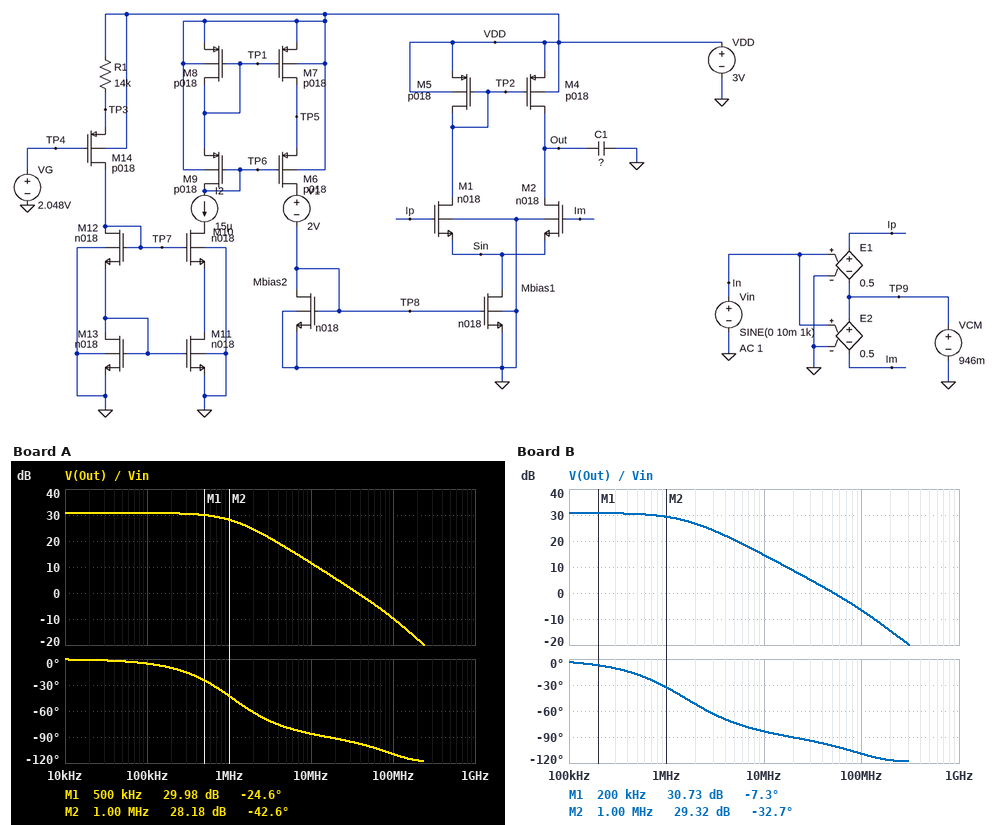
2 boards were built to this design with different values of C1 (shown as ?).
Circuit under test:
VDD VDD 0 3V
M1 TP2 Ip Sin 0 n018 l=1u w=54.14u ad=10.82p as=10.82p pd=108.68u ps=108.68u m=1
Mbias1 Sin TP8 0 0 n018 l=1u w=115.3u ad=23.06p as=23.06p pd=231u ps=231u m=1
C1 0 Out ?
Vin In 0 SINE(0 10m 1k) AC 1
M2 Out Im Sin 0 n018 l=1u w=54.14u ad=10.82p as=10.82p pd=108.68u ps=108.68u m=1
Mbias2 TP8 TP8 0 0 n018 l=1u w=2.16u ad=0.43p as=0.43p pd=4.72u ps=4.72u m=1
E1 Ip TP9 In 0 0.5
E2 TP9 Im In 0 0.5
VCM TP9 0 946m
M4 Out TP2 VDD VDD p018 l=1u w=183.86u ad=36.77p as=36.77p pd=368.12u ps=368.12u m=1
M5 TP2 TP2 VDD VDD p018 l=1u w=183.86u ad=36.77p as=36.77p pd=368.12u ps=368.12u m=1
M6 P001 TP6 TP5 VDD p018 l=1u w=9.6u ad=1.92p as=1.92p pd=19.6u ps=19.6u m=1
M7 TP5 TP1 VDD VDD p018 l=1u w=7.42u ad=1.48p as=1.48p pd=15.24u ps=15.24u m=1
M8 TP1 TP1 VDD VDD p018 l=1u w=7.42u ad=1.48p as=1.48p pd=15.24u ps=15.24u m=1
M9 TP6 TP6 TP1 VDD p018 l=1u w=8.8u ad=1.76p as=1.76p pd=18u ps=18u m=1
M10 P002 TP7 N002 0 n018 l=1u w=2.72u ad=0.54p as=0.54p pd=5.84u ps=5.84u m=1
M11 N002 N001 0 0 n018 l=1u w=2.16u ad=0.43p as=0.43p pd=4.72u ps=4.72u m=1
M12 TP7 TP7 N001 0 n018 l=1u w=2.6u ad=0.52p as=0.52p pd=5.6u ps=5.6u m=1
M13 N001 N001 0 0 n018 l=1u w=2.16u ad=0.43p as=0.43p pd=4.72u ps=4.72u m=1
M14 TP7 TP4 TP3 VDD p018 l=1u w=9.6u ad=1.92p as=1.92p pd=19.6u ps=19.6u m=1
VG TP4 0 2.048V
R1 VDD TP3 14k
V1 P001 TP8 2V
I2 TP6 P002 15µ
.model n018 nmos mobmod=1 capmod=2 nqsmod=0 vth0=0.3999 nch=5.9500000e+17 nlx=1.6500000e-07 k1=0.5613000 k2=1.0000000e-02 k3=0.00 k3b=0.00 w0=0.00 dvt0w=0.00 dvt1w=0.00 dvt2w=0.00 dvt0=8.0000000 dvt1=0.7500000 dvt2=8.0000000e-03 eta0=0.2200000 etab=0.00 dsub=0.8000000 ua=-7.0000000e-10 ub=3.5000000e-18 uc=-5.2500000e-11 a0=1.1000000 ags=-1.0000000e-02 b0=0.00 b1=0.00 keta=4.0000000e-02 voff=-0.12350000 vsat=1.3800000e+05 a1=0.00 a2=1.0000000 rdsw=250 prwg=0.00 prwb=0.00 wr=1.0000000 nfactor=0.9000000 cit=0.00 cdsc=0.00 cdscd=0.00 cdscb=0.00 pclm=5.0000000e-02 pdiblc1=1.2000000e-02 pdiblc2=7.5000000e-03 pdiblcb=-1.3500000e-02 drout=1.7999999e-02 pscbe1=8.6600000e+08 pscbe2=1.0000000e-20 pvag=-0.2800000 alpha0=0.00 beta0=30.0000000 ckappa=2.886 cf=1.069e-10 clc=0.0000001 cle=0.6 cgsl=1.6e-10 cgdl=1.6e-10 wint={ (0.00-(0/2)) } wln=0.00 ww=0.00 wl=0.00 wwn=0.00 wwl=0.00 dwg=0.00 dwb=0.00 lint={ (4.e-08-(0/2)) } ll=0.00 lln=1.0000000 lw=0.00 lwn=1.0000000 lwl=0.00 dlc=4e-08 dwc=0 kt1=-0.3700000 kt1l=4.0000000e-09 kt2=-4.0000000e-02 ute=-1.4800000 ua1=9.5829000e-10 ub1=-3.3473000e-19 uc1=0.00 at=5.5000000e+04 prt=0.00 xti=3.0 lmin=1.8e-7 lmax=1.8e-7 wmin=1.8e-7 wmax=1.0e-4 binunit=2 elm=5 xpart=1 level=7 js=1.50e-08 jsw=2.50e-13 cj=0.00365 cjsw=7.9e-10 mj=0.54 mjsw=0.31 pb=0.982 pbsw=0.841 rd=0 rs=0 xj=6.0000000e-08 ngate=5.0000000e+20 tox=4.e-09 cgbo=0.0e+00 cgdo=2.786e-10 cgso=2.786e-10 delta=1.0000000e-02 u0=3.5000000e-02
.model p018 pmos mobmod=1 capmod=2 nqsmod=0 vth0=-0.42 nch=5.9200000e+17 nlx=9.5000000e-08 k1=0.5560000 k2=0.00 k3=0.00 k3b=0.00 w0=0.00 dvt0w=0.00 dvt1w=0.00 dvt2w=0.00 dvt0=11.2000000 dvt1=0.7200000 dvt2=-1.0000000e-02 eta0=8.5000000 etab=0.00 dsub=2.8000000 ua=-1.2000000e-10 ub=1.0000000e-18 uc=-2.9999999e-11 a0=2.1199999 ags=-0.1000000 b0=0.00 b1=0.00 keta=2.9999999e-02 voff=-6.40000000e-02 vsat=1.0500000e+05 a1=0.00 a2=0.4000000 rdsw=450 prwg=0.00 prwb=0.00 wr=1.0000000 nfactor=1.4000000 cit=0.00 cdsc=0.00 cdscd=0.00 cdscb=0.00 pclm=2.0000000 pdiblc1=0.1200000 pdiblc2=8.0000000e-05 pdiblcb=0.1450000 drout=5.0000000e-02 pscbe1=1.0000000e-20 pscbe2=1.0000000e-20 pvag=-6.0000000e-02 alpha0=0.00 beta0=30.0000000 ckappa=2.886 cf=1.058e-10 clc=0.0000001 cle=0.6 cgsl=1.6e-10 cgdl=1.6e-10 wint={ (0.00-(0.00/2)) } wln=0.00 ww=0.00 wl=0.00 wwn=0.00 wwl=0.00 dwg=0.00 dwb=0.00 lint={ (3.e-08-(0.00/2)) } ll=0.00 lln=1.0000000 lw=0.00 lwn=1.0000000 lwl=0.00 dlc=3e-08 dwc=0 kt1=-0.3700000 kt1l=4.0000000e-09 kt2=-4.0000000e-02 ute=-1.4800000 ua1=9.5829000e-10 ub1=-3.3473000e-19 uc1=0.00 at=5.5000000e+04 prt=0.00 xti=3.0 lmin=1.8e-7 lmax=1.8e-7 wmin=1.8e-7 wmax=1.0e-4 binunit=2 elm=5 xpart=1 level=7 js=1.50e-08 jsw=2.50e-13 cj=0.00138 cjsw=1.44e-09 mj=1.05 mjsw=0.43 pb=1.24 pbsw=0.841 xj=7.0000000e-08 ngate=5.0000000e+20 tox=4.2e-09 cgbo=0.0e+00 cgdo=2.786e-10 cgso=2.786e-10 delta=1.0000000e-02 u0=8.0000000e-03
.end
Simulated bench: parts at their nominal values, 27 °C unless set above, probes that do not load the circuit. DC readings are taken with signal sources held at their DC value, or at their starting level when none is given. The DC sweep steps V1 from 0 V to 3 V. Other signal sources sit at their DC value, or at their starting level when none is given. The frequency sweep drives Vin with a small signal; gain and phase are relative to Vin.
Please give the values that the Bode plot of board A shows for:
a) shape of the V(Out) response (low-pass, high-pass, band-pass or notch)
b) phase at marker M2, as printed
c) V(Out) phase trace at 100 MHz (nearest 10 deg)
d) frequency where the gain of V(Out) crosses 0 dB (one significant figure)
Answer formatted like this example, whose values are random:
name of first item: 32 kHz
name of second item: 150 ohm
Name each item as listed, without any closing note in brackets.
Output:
shape of the V(Out) response: low-pass
phase at marker M2, as printed: -42.6 deg
V(Out) phase trace at 100 MHz: -110 deg
frequency where the gain of V(Out) crosses 0 dB: 40 MHz
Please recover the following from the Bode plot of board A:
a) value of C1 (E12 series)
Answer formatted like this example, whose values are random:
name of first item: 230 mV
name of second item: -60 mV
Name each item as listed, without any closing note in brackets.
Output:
value of C1: 10 pF
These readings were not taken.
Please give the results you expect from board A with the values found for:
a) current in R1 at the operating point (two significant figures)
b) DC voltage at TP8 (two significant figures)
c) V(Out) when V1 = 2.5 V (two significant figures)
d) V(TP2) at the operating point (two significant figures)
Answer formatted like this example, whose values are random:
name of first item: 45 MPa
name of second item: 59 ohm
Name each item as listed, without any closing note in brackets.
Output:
current in R1 at the operating point: 16 µA
DC voltage at TP8: 680 mV
V(Out) when V1 = 2.5 V: 2.5 V
V(TP2) at the operating point: 2.2 V
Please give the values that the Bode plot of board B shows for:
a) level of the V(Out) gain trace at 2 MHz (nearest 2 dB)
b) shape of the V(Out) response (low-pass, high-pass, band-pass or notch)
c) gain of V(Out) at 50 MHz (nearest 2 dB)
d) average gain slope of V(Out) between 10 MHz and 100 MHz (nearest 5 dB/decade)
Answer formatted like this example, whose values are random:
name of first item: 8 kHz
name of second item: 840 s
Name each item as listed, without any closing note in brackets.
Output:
level of the V(Out) gain trace at 2 MHz: 26 dB
shape of the V(Out) response: low-pass
gain of V(Out) at 50 MHz: 0 dB
average gain slope of V(Out) between 10 MHz and 100 MHz: -20 dB/decade
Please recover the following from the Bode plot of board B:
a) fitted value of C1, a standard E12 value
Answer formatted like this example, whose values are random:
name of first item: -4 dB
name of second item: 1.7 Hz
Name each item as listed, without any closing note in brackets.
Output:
fitted value of C1, a standard E12 value: 6.8 pF
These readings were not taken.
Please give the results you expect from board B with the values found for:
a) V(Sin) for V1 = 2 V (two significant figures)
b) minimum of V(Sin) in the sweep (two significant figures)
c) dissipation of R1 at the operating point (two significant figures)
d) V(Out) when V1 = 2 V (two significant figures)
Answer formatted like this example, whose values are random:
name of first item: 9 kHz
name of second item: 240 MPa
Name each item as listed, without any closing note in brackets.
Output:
V(Sin) for V1 = 2 V: 240 mV
minimum of V(Sin) in the sweep: 230 mV
dissipation of R1 at the operating point: 3.5 µW
V(Out) when V1 = 2 V: 2.2 V
